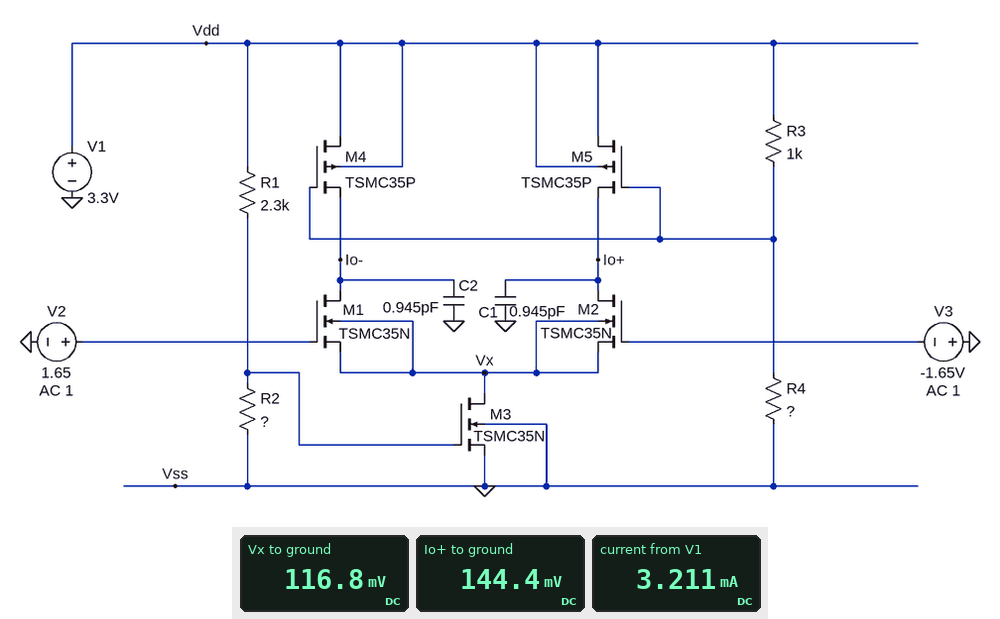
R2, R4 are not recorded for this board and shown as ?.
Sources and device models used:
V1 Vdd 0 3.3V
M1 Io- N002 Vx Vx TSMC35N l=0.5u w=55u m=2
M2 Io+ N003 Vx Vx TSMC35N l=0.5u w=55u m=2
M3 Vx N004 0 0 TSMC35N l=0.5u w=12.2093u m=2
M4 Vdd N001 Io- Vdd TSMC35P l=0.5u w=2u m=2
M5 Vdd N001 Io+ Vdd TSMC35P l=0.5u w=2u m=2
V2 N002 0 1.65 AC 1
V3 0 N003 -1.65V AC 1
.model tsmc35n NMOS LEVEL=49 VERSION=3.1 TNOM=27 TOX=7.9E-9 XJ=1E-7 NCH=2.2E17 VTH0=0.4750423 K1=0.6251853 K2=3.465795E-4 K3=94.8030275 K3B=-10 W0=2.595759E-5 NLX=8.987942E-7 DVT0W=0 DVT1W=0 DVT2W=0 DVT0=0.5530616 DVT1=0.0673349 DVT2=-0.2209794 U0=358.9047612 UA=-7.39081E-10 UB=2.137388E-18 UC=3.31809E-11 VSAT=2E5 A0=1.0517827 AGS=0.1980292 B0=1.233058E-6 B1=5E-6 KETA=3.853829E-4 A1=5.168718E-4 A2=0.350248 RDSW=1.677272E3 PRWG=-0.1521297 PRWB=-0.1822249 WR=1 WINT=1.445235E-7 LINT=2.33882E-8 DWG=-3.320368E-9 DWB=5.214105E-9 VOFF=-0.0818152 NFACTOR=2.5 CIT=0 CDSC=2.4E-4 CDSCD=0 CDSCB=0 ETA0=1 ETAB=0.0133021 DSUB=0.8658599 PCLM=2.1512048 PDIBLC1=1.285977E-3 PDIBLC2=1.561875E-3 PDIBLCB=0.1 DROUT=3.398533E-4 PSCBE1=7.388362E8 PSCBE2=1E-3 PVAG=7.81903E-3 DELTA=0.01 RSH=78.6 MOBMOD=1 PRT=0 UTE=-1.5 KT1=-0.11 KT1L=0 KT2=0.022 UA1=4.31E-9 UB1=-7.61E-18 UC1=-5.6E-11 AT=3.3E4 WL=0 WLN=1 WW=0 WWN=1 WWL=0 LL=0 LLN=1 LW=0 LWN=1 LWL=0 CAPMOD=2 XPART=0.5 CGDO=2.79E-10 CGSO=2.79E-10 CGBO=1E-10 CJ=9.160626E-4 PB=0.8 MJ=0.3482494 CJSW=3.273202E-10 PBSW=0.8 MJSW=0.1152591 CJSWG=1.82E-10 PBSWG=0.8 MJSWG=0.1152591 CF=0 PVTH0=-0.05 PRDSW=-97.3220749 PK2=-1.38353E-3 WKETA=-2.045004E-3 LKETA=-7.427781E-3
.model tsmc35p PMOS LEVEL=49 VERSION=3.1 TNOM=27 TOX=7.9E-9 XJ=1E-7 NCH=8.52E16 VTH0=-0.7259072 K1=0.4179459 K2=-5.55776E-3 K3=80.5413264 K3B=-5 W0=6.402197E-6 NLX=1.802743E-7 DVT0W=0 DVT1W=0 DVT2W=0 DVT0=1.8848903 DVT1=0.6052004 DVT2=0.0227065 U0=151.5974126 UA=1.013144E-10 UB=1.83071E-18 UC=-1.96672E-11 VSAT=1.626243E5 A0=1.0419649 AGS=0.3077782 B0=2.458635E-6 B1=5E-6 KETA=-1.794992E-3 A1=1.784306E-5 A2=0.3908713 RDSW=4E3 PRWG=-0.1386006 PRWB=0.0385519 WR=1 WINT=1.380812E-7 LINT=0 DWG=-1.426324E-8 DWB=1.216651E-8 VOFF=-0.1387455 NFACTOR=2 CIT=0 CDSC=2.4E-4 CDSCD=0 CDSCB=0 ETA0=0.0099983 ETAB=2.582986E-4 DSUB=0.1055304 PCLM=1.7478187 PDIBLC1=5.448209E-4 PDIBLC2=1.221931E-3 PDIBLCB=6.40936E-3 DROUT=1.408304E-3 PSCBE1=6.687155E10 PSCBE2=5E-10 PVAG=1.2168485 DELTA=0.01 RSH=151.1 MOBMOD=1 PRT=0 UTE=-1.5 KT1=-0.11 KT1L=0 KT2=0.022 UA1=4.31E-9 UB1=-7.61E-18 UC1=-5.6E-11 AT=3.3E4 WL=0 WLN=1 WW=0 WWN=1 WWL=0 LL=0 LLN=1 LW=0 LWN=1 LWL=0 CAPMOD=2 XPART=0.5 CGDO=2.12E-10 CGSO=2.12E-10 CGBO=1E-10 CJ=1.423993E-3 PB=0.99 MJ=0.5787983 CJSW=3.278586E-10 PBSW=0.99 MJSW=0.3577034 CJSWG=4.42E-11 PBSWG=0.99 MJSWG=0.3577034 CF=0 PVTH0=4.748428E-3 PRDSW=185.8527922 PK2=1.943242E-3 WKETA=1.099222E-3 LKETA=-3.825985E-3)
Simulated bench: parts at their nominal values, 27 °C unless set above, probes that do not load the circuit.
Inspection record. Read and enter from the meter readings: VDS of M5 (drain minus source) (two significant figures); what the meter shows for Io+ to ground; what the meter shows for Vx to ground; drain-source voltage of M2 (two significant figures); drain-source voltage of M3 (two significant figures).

3.2 V
144.4 mV
116.8 mV
28 mV
120 mV
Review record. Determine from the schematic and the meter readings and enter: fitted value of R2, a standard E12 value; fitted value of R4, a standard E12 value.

2.7 kΩ
560 Ω
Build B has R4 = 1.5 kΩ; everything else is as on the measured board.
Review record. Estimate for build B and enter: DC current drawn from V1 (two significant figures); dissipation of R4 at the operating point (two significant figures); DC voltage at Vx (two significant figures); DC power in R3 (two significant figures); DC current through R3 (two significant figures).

2.1 mA
2.6 mW
26 mV
1.7 mW
1.3 mA
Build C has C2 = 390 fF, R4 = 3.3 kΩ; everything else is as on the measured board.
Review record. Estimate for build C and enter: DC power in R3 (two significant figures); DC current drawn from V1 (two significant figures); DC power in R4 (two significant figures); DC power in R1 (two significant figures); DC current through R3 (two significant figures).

590 µW
1.4 mA
1.9 mW
1.0 mW
770 µA
